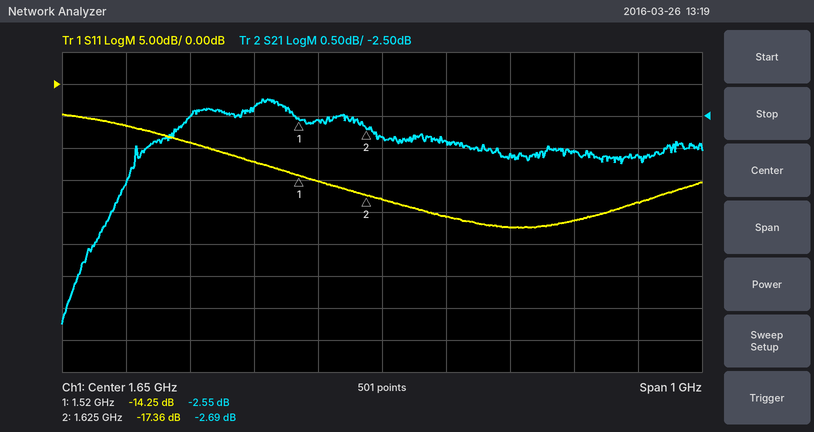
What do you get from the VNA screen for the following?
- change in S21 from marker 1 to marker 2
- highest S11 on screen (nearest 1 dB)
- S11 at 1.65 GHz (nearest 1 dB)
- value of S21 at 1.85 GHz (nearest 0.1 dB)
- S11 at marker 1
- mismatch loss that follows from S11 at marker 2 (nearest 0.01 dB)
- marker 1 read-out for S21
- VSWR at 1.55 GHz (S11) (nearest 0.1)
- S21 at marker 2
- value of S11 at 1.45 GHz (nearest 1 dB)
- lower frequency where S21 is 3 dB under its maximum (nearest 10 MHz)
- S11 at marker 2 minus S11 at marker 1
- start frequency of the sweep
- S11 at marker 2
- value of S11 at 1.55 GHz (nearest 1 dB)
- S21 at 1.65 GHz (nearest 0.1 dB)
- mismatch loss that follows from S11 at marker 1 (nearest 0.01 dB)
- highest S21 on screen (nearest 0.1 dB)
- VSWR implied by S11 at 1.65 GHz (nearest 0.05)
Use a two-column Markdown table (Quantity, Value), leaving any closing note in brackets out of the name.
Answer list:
| Quantity | Value |
|---|---|
| change in S21 from marker 1 to marker 2 | -0.14 dB |
| highest S11 on screen | -5 dB |
| S11 at 1.65 GHz | -18 dB |
| value of S21 at 1.85 GHz | -3.1 dB |
| S11 at marker 1 | -14.25 dB |
| mismatch loss that follows from S11 at marker 2 | 0.08 dB |
| marker 1 read-out for S21 | -2.55 dB |
| VSWR at 1.55 GHz (S11) | 1.4 |
| S21 at marker 2 | -2.69 dB |
| value of S11 at 1.45 GHz | -12 dB |
| lower frequency where S21 is 3 dB under its maximum | 1.17 GHz |
| S11 at marker 2 minus S11 at marker 1 | -3.11 dB |
| start frequency of the sweep | 1.15 GHz |
| S11 at marker 2 | -17.36 dB |
| value of S11 at 1.55 GHz | -15 dB |
| S21 at 1.65 GHz | -2.8 dB |
| mismatch loss that follows from S11 at marker 1 | 0.17 dB |
| highest S21 on screen | -2.2 dB |
| VSWR implied by S11 at 1.65 GHz | 1.30 |
